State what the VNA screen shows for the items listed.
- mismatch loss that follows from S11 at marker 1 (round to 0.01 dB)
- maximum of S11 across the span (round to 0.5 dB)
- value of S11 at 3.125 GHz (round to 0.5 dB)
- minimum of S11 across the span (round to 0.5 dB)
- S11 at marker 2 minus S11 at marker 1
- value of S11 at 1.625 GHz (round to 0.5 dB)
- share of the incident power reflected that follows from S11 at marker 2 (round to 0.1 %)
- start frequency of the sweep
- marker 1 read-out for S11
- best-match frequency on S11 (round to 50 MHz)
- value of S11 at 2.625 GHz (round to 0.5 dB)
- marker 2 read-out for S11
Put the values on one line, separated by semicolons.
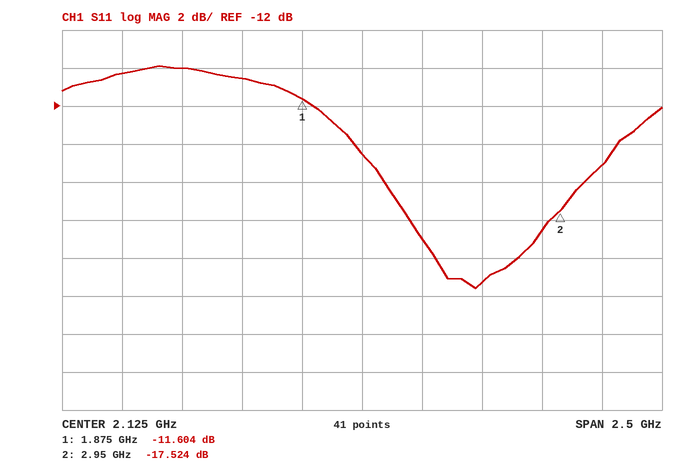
0.31 dB; -10.0 dB; -15.0 dB; -21.5 dB; -5.920 dB; -10.5 dB; 1.8 %; 875 MHz; -11.604 dB; 2.60 GHz; -21.5 dB; -17.524 dB
